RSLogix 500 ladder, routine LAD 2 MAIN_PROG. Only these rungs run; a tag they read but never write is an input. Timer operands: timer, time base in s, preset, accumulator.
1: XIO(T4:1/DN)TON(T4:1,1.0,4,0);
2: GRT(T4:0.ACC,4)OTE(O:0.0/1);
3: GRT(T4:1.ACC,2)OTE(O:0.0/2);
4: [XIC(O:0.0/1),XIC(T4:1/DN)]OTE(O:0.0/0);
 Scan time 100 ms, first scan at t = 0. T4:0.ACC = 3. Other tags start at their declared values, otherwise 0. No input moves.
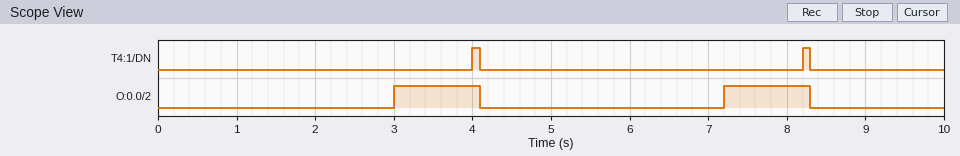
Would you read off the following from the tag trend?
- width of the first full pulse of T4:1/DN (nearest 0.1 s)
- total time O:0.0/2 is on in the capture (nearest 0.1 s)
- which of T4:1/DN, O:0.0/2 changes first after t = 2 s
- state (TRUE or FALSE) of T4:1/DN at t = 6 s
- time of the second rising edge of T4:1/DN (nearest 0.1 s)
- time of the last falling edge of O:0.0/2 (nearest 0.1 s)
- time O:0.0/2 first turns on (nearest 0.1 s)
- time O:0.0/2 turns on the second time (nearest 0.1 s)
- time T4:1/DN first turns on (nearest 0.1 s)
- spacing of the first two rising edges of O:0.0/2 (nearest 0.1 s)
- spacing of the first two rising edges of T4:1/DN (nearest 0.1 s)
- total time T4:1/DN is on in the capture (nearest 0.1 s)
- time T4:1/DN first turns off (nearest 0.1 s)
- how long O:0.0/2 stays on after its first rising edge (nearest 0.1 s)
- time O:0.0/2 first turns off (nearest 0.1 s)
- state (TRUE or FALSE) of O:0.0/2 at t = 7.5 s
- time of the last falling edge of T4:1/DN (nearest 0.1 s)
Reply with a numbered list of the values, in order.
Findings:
1. 0.1 s
2. 2.2 s
3. O:0.0/2
4. FALSE
5. 8.2 s
6. 8.3 s
7. 3.0 s
8. 7.2 s
9. 4.0 s
10. 4.2 s
11. 4.2 s
12. 0.2 s
13. 4.1 s
14. 1.1 s
15. 4.1 s
16. TRUE
17. 8.3 s
